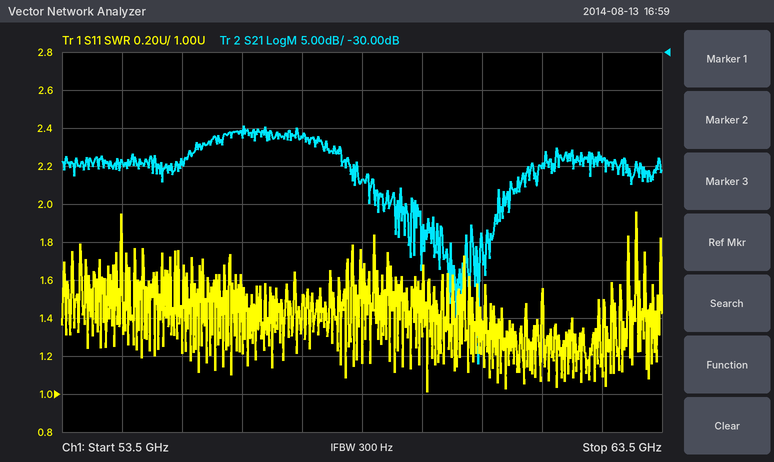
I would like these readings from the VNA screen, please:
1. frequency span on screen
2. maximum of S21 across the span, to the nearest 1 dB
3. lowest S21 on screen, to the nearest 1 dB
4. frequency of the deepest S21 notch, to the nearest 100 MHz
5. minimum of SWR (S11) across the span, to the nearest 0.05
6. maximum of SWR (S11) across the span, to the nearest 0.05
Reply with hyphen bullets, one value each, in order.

- 10 GHz
- -40 dB
- -71 dB
- 60.4 GHz
- 1.00
- 1.95
